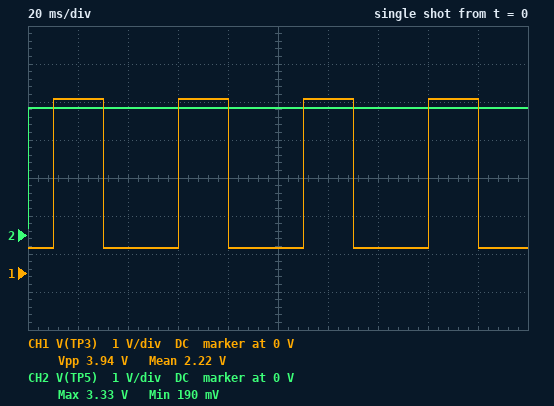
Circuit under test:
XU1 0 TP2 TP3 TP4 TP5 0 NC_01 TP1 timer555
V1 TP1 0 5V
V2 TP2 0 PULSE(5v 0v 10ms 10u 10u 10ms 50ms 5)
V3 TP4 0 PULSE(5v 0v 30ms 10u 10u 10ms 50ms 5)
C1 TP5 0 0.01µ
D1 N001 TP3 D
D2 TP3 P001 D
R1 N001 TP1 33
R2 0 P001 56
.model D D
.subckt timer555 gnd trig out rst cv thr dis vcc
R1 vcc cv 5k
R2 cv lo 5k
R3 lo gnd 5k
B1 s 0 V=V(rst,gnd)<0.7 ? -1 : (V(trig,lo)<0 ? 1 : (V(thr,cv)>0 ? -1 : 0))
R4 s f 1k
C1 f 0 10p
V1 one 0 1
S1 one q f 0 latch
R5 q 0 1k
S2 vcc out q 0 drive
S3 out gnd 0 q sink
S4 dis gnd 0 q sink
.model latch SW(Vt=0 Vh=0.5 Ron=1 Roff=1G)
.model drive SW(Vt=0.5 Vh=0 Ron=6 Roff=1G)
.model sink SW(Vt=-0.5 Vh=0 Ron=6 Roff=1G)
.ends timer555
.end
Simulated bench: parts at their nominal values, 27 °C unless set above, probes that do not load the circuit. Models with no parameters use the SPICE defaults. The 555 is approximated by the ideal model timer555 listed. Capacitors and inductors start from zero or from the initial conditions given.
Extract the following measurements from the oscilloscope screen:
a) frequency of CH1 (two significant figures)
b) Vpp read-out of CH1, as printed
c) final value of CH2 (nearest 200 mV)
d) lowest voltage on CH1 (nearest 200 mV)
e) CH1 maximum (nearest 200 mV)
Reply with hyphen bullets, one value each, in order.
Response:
- 20 Hz
- 3.94 V
- 3.4 V
- 600 mV
- 4.6 V
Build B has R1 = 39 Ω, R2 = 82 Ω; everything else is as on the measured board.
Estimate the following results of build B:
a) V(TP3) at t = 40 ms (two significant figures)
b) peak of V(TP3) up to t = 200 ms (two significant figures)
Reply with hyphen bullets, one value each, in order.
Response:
- 560 mV
- 4.7 V
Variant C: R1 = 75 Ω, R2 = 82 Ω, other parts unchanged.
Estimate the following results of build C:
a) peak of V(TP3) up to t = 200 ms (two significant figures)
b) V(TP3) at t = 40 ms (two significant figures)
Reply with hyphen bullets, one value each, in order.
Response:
- 4.7 V
- 310 mV
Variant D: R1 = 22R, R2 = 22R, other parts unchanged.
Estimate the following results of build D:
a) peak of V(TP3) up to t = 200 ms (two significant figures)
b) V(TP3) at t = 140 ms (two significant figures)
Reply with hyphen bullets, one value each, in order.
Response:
- 4.1 V
- 870 mV
